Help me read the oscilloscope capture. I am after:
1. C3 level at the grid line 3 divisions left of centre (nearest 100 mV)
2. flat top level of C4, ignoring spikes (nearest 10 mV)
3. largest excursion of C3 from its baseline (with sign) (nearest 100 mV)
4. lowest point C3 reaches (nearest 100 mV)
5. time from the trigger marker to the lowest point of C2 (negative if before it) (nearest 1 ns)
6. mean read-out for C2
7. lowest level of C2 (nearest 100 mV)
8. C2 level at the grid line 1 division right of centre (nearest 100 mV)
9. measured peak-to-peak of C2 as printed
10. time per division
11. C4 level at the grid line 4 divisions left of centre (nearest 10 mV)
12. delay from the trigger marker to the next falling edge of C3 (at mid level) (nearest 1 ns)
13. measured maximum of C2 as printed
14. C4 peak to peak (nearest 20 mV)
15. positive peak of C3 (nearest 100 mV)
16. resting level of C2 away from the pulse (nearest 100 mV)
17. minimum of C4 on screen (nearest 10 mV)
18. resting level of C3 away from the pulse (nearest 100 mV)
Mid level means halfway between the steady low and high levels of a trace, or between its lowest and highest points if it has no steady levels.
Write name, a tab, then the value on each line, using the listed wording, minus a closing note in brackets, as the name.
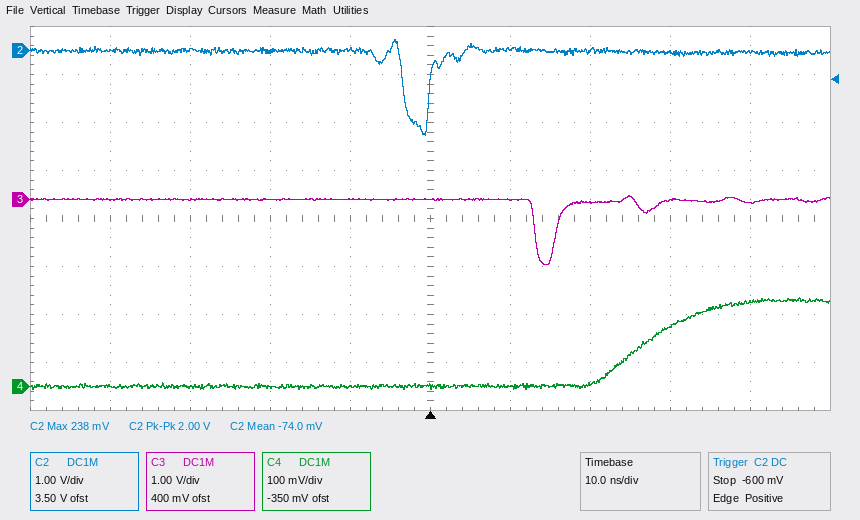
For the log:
C3 level at the grid line 3 divisions left of centre	0.0 V
flat top level of C4, ignoring spikes	180 mV
largest excursion of C3 from its baseline (with sign)	-1.4 V
lowest point C3 reaches	-1.4 V
time from the trigger marker to the lowest point of C2 (negative if before it)	-1 ns
mean read-out for C2	-74.0 mV
lowest level of C2	-1.8 V
C2 level at the grid line 1 division right of centre	0.0 V
measured peak-to-peak of C2 as printed	2.00 V
time per division	10 ns
C4 level at the grid line 4 divisions left of centre	0 mV
delay from the trigger marker to the next falling edge of C3 (at mid level)	13 ns
measured maximum of C2 as printed	238 mV
C4 peak to peak	200 mV
positive peak of C3	100 mV
resting level of C2 away from the pulse	0.0 V
minimum of C4 on screen	-10 mV
resting level of C3 away from the pulse	0.0 V
